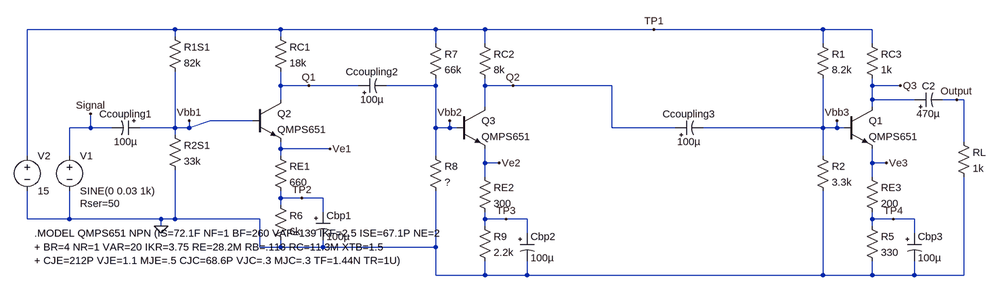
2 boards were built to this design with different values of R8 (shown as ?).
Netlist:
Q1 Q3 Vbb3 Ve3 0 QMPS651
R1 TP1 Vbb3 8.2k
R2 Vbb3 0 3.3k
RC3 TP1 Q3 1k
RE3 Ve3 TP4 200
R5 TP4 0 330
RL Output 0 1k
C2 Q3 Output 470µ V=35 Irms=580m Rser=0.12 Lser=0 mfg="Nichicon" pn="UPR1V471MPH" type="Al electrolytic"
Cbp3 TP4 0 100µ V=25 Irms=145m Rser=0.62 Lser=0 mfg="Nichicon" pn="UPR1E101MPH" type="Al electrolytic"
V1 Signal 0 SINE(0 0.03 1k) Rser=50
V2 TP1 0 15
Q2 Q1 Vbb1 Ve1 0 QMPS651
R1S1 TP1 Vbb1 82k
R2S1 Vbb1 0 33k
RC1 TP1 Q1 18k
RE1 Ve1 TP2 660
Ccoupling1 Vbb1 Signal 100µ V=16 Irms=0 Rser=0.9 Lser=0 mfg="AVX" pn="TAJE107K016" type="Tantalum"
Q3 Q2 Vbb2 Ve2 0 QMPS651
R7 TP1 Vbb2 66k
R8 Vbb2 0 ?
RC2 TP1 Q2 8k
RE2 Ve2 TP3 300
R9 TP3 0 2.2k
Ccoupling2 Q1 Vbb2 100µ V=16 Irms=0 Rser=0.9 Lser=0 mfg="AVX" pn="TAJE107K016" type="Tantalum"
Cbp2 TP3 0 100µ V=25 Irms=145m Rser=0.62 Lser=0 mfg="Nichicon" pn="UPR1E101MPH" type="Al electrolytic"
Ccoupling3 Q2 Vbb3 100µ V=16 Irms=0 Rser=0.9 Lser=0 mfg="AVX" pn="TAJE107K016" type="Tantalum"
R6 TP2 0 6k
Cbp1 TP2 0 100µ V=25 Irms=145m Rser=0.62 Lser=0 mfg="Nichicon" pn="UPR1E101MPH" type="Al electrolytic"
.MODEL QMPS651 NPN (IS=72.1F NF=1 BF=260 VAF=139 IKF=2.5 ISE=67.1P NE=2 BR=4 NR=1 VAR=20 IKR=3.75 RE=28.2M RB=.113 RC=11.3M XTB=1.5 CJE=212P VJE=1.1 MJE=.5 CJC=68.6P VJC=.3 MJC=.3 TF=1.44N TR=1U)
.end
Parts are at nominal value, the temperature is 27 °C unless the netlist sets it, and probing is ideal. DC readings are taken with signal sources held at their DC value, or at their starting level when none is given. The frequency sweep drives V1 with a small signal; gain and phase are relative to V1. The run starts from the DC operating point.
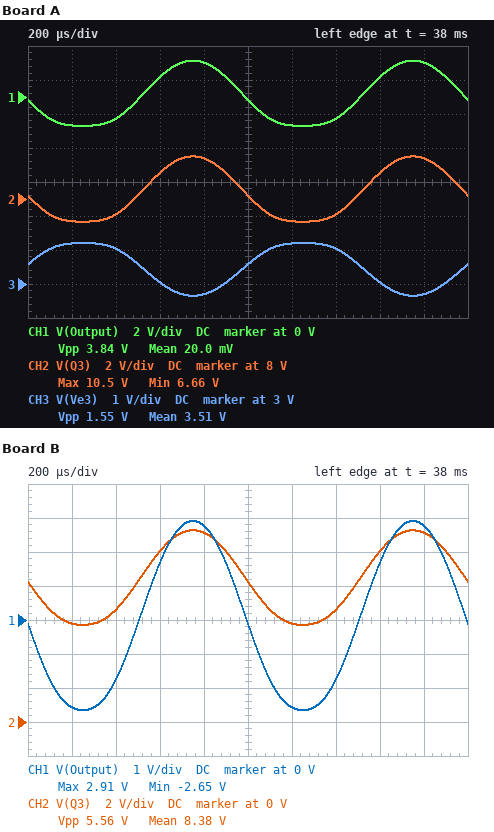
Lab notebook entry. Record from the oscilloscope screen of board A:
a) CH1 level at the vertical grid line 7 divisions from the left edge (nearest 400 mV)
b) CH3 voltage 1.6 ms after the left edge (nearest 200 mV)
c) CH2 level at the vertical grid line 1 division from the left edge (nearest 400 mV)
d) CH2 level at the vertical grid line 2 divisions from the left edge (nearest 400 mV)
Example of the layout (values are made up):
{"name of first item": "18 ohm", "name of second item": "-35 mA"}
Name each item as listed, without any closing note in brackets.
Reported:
{"CH1 level at the vertical grid line 7 divisions from the left edge": "-1.2 V", "CH3 voltage 1.6 ms after the left edge": "3.0 V", "CH2 level at the vertical grid line 1 division from the left edge": "6.8 V", "CH2 level at the vertical grid line 2 divisions from the left edge": "7.2 V"}
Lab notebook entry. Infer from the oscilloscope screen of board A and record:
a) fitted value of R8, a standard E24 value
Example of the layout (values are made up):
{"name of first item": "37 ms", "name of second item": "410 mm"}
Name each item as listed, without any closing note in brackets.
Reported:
{"fitted value of R8, a standard E24 value": "8.2 kΩ"}
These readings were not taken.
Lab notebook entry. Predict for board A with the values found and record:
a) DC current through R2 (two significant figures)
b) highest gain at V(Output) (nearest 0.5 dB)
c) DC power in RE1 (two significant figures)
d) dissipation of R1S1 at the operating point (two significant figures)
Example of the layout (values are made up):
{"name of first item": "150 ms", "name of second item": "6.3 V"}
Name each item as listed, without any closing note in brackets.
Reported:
{"DC current through R2": "1.3 mA", "highest gain at V(Output)": "37.0 dB", "DC power in RE1": "190 µW", "dissipation of R1S1 at the operating point": "1.4 mW"}
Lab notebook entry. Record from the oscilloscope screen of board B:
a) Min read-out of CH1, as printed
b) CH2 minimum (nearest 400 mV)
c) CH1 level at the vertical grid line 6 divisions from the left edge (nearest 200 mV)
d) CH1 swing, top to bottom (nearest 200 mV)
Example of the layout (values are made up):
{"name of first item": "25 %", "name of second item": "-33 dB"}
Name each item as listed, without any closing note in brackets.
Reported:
{"Min read-out of CH1, as printed": "-2.65 V", "CH2 minimum": "5.6 V", "CH1 level at the vertical grid line 6 divisions from the left edge": "-2.6 V", "CH1 swing, top to bottom": "5.6 V"}
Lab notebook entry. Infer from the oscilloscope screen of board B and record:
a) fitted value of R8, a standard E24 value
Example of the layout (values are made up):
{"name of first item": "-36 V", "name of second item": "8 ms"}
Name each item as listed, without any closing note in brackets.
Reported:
{"fitted value of R8, a standard E24 value": "13 kΩ"}
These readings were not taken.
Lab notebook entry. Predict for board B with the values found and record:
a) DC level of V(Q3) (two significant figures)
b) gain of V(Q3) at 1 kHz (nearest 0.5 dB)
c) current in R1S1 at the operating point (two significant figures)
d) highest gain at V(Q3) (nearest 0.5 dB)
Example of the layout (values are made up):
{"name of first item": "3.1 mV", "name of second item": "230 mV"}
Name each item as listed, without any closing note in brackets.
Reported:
{"DC level of V(Q3)": "8.4 V", "gain of V(Q3) at 1 kHz": "40.0 dB", "current in R1S1 at the operating point": "130 µA", "highest gain at V(Q3)": "40.0 dB"}
